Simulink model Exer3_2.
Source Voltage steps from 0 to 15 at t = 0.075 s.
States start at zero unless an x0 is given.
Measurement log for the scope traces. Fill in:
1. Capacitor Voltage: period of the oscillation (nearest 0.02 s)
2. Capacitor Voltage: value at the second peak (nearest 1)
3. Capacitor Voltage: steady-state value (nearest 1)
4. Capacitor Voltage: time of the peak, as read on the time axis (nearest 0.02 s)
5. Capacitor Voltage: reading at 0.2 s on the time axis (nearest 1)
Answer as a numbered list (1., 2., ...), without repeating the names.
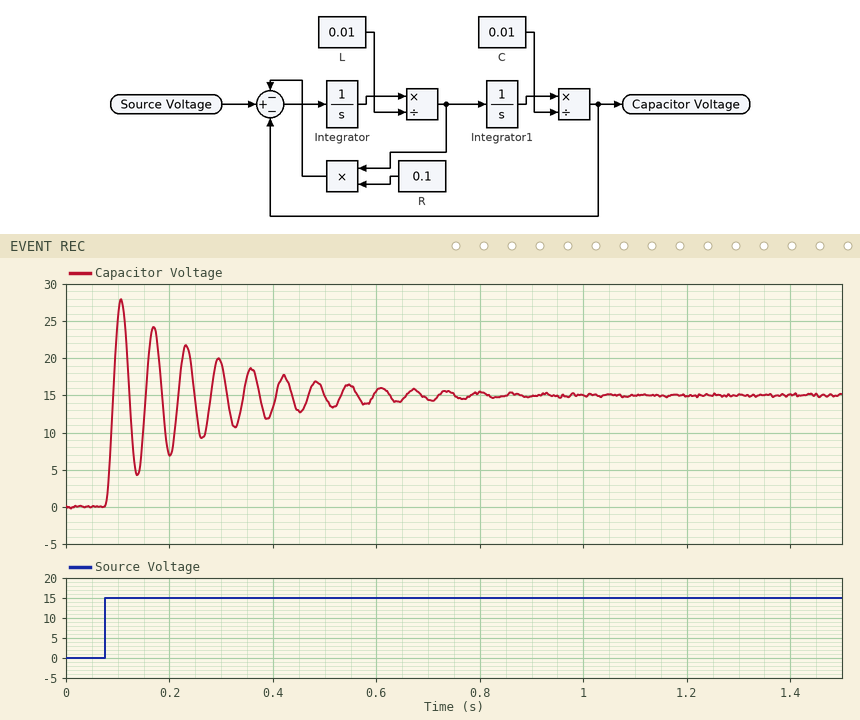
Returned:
1. 0.06 s
2. 24
3. 15
4. 0.10 s
5. 7
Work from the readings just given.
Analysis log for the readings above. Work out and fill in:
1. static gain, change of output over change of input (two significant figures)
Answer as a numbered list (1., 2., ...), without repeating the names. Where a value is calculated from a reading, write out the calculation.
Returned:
1. (15 - 0) / (15 - 0) = 1.0
